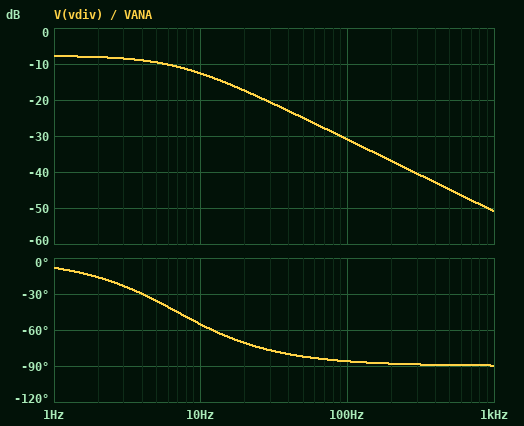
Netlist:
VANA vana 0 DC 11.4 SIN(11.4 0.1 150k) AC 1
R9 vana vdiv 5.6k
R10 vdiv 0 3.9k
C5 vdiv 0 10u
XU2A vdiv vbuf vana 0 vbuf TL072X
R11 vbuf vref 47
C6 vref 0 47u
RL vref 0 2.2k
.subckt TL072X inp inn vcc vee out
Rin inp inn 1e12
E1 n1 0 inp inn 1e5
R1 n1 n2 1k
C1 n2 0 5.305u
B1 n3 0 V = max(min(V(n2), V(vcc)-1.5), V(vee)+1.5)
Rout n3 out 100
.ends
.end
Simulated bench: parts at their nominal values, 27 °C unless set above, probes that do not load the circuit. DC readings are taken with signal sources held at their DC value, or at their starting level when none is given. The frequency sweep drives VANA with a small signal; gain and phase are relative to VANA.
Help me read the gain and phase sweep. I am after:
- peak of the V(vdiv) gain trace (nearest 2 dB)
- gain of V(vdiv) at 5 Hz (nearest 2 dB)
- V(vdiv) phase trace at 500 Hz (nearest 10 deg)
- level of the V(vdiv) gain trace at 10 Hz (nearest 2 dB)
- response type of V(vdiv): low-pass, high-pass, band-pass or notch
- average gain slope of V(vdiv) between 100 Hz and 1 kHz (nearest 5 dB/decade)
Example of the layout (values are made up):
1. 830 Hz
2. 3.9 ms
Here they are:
1. -8 dB
2. -10 dB
3. -90 deg
4. -12 dB
5. low-pass
6. -20 dB/decade
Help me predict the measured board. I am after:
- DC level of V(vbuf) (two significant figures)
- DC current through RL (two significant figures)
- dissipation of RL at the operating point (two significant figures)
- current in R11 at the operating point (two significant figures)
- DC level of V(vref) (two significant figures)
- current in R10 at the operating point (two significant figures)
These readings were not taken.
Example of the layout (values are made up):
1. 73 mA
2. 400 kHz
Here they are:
1. 4.7 V
2. 2.1 mA
3. 9.5 mW
4. 2.1 mA
5. 4.6 V
6. 1.2 mA
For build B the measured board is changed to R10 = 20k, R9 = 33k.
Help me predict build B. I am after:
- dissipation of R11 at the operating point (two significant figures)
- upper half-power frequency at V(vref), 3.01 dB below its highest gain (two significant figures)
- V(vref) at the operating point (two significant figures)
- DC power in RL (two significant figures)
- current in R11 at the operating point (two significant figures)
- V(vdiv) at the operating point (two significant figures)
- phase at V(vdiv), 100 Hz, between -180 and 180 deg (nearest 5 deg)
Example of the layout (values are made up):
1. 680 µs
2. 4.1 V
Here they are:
1. 170 µW
2. 1.3 Hz
3. 4.2 V
4. 8.1 mW
5. 1.9 mA
6. 4.3 V
7. -90 deg
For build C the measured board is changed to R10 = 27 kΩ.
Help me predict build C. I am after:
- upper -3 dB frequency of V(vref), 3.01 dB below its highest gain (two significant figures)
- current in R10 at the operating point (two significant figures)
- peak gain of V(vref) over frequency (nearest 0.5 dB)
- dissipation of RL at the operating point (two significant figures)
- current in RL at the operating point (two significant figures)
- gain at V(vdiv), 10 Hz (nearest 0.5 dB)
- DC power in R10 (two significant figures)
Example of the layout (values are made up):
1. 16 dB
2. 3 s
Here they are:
1. 3.4 Hz
2. 350 µA
3. -2.0 dB
4. 39 mW
5. 4.2 mA
6. -11.5 dB
7. 3.3 mW
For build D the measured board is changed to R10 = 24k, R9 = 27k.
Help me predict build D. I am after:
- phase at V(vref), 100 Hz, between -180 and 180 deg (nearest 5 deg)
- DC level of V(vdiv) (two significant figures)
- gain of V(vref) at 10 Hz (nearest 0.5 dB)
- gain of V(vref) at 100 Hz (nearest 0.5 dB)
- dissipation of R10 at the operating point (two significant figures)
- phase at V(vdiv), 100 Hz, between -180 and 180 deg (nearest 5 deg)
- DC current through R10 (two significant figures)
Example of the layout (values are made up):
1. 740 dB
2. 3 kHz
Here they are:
1. -145 deg
2. 5.4 V
3. -25.0 dB
4. -49.5 dB
5. 1.2 mW
6. -90 deg
7. 220 µA
